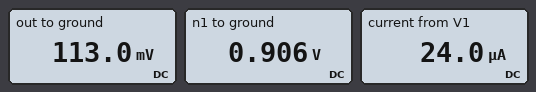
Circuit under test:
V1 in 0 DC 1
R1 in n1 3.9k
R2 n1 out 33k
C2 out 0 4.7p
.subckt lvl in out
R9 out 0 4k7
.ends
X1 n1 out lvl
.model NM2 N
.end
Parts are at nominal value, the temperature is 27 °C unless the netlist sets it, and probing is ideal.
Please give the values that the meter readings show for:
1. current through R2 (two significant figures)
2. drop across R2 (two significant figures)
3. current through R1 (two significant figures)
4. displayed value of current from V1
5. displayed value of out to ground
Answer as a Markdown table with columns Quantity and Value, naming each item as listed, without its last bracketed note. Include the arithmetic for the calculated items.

| Quantity | Value |
|---|---|
| current through R2 | (906 mV - 113 mV) / 33 kΩ = 24 µA |
| drop across R2 | 906 mV - 113 mV = 790 mV |
| current through R1 | (1 V - 906 mV) / 3.9 kΩ = 24 µA |
| displayed value of current from V1 | 24.0 µA |
| displayed value of out to ground | 113.0 mV |
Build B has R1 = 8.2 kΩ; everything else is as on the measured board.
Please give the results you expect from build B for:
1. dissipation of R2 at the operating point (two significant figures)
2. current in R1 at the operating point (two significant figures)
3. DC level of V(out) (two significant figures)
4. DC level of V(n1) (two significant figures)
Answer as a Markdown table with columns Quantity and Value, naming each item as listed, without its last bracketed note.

| Quantity | Value |
|---|---|
| dissipation of R2 at the operating point | 16 µW |
| current in R1 at the operating point | 22 µA |
| DC level of V(out) | 100 mV |
| DC level of V(n1) | 820 mV |
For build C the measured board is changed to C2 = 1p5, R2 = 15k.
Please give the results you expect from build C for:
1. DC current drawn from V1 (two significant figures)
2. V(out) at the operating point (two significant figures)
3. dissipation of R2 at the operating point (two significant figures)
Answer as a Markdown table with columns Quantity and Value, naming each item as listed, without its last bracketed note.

| Quantity | Value |
|---|---|
| DC current drawn from V1 | 42 µA |
| V(out) at the operating point | 200 mV |
| dissipation of R2 at the operating point | 27 µW |
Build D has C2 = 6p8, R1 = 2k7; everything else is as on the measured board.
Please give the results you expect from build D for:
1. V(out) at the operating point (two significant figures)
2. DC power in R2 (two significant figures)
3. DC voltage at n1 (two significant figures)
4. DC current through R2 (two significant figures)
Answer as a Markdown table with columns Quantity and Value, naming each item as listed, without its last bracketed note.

| Quantity | Value |
|---|---|
| V(out) at the operating point | 120 mV |
| DC power in R2 | 20 µW |
| DC voltage at n1 | 930 mV |
| DC current through R2 | 25 µA |
